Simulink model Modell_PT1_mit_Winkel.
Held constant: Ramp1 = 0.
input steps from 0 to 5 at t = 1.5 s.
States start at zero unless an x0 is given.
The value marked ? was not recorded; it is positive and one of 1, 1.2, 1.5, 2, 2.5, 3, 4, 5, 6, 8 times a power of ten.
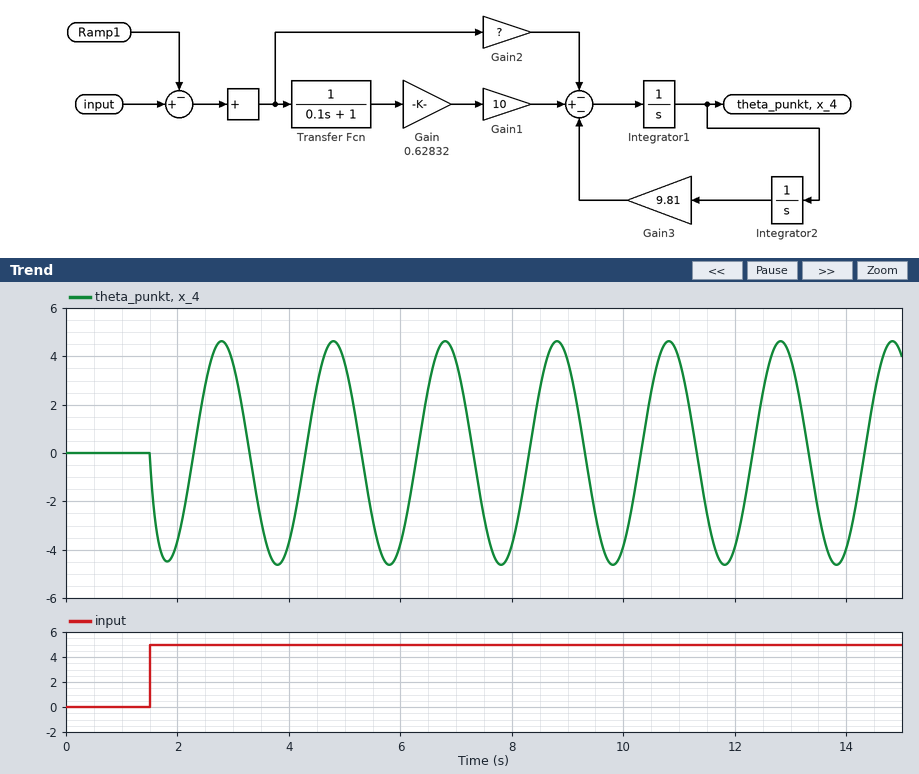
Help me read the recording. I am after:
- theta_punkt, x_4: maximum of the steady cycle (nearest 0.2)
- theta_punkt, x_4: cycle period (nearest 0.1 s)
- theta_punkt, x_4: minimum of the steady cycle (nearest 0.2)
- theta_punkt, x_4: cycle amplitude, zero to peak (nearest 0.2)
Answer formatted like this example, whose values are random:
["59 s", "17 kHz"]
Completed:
["4.6", "2.0 s", "-4.6", "4.6"]
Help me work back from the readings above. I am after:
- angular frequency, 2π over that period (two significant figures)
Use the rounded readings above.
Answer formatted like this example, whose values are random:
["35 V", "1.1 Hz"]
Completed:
["3.1 rad/s"]
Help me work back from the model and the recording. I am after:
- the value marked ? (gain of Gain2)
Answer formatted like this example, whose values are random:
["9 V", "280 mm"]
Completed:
["8"]
